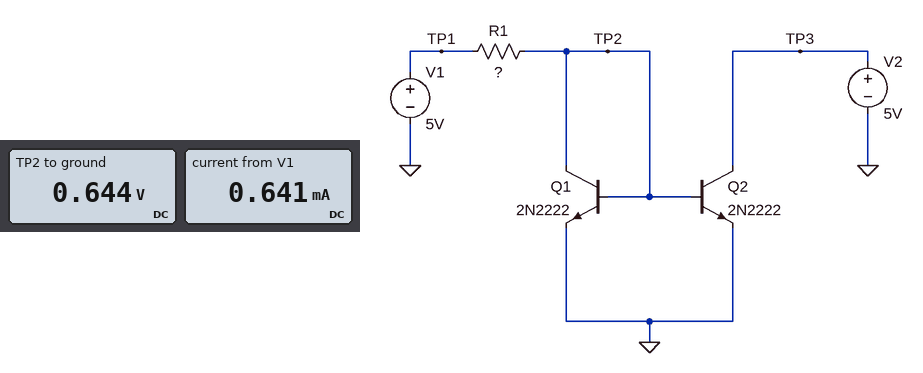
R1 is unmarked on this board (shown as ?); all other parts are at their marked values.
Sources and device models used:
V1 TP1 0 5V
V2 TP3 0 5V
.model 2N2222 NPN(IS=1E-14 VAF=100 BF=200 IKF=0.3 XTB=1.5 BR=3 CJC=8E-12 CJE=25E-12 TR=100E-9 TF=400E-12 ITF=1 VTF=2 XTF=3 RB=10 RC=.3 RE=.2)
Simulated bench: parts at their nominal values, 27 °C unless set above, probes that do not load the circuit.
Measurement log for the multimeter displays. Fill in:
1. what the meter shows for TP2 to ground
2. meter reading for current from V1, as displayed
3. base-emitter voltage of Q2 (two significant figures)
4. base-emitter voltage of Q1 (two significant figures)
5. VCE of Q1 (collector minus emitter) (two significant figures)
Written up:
0.644 V
0.641 mA
640 mV
640 mV
640 mV
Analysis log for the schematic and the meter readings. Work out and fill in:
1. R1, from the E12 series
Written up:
6.8 kΩ
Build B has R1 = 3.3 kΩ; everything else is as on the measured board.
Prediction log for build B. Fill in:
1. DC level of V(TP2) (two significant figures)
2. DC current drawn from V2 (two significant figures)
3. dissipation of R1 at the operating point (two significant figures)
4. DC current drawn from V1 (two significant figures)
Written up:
660 mV
1.4 mA
5.7 mW
1.3 mA
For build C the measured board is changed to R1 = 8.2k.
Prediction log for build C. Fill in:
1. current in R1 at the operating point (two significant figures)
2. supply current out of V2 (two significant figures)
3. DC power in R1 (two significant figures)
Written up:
530 µA
550 µA
2.3 mW
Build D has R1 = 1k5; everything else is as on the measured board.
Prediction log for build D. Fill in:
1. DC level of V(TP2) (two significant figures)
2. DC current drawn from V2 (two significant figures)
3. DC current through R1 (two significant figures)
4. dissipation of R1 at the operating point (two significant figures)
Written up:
680 mV
3.0 mA
2.9 mA
12 mW
